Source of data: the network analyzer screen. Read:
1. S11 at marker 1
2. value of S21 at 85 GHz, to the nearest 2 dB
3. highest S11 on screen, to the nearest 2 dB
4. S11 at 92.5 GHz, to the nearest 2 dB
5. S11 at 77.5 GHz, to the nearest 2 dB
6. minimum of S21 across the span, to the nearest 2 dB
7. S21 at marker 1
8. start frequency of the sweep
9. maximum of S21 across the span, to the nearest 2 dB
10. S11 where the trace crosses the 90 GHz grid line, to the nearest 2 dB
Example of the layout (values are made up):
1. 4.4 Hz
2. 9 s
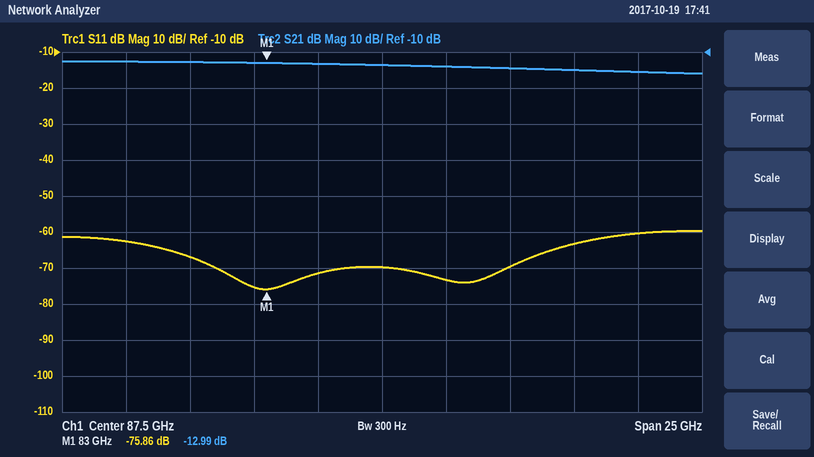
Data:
1. -75.86 dB
2. -14 dB
3. -60 dB
4. -70 dB
5. -62 dB
6. -16 dB
7. -12.99 dB
8. 75 GHz
9. -12 dB
10. -74 dB
